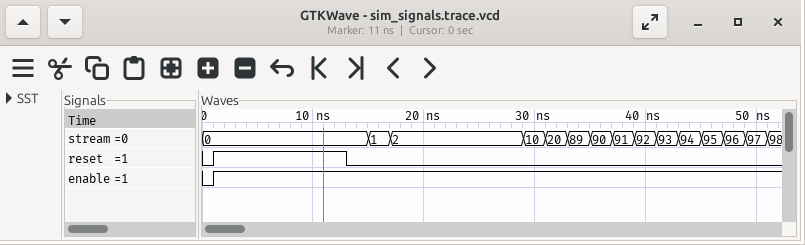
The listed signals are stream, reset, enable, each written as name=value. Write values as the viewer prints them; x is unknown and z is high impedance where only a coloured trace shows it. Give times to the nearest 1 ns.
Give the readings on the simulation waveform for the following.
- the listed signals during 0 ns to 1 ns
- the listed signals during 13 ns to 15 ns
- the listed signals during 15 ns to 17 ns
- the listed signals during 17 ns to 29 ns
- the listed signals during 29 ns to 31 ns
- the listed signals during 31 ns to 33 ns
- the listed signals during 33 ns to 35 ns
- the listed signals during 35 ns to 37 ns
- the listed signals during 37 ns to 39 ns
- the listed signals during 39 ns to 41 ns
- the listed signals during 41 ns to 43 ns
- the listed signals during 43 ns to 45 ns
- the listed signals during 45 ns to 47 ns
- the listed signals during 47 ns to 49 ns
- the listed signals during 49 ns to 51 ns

stream=0, reset=0, enable=0
stream=0, reset=0, enable=1
stream=1, reset=0, enable=1
stream=2, reset=0, enable=1
stream=10, reset=0, enable=1
stream=20, reset=0, enable=1
stream=89, reset=0, enable=1
stream=90, reset=0, enable=1
stream=91, reset=0, enable=1
stream=92, reset=0, enable=1
stream=93, reset=0, enable=1
stream=94, reset=0, enable=1
stream=95, reset=0, enable=1
stream=96, reset=0, enable=1
stream=97, reset=0, enable=1
